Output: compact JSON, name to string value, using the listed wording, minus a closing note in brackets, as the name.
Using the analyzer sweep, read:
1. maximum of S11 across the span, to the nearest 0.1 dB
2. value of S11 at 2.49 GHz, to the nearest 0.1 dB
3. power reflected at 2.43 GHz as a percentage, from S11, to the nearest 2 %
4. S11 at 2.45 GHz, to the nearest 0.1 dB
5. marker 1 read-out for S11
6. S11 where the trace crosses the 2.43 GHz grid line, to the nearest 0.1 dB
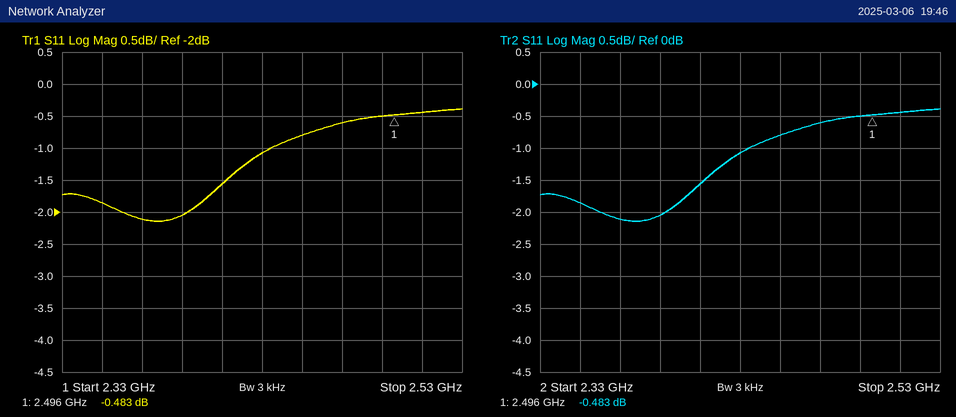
{"maximum of S11 across the span, to the nearest 0.1 dB": "-0.4 dB", "value of S11 at 2.49 GHz, to the nearest 0.1 dB": "-0.5 dB", "power reflected at 2.43 GHz as a percentage, from S11, to the nearest 2 %": "78 %", "S11 at 2.45 GHz, to the nearest 0.1 dB": "-0.8 dB", "marker 1 read-out for S11": "-0.483 dB", "S11 where the trace crosses the 2.43 GHz grid line, to the nearest 0.1 dB": "-1.1 dB"}
